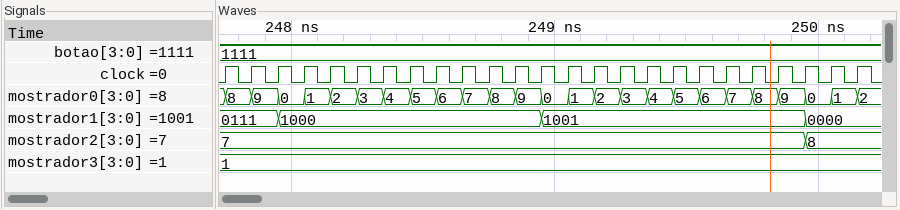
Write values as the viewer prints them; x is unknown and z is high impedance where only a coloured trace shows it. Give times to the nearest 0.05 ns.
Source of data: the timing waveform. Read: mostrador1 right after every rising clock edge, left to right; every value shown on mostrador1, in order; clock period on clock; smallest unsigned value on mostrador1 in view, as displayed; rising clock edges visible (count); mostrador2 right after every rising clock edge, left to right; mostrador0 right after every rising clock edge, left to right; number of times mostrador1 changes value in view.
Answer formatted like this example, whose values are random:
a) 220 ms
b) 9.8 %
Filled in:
a) 0111, 0111, 1000, 1000, 1000, 1000, 1000, 1000, 1000, 1000, 1000, 1000, 1001, 1001, 1001, 1001, 1001, 1001, 1001, 1001, 1001, 1001, 0000, 0000, 0000
b) 0111, 1000, 1001, 0000
c) 0.1 ns
d) 0000
e) 25
f) 7, 7, 7, 7, 7, 7, 7, 7, 7, 7, 7, 7, 7, 7, 7, 7, 7, 7, 7, 7, 7, 7, 8, 8, 8
g) 8, 9, 0, 1, 2, 3, 4, 5, 6, 7, 8, 9, 0, 1, 2, 3, 4, 5, 6, 7, 8, 9, 0, 1, 2
h) 3
